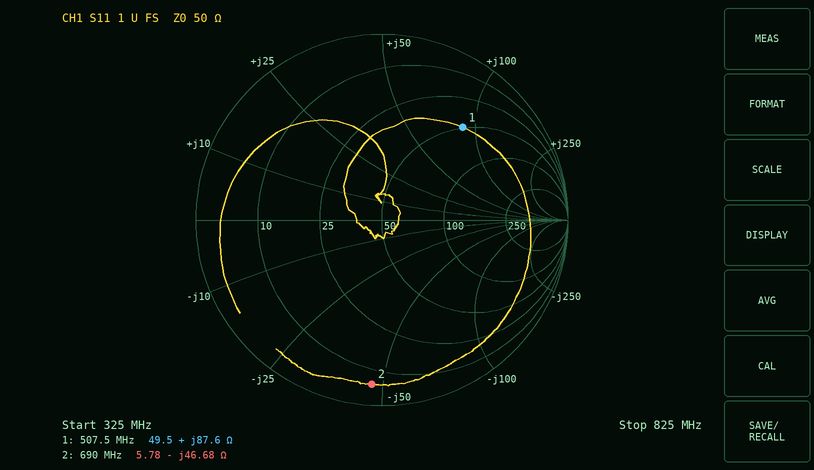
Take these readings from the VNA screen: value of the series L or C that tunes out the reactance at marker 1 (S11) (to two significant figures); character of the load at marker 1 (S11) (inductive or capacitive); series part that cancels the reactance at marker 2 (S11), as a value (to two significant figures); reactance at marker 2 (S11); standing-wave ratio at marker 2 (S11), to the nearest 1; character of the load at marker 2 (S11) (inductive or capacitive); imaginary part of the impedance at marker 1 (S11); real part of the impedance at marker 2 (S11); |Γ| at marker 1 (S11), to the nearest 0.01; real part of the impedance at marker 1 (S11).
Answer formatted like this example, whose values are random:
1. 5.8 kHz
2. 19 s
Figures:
1. 3.6 pF
2. inductive
3. 11 nH
4. -46.68 Ω
5. 16
6. capacitive
7. +87.6 Ω
8. 5.78 Ω
9. 0.66
10. 49.5 Ω
